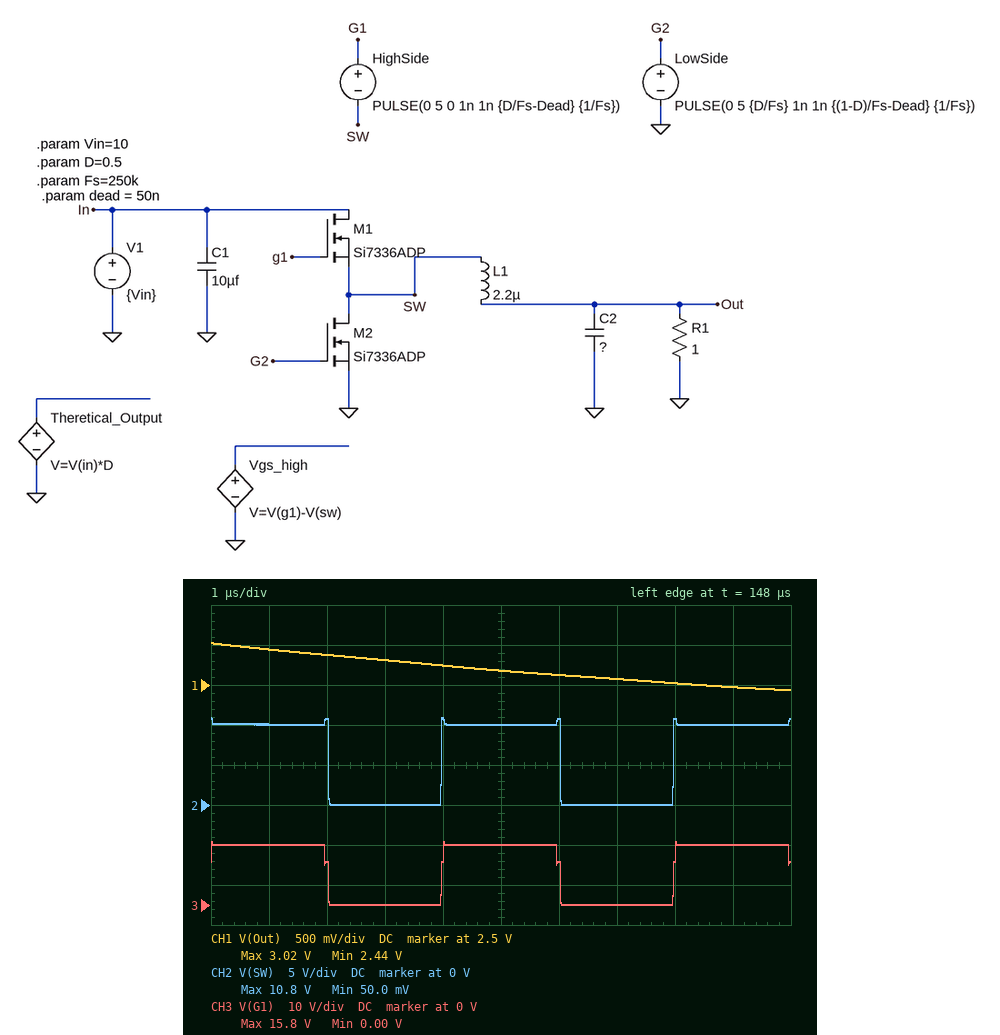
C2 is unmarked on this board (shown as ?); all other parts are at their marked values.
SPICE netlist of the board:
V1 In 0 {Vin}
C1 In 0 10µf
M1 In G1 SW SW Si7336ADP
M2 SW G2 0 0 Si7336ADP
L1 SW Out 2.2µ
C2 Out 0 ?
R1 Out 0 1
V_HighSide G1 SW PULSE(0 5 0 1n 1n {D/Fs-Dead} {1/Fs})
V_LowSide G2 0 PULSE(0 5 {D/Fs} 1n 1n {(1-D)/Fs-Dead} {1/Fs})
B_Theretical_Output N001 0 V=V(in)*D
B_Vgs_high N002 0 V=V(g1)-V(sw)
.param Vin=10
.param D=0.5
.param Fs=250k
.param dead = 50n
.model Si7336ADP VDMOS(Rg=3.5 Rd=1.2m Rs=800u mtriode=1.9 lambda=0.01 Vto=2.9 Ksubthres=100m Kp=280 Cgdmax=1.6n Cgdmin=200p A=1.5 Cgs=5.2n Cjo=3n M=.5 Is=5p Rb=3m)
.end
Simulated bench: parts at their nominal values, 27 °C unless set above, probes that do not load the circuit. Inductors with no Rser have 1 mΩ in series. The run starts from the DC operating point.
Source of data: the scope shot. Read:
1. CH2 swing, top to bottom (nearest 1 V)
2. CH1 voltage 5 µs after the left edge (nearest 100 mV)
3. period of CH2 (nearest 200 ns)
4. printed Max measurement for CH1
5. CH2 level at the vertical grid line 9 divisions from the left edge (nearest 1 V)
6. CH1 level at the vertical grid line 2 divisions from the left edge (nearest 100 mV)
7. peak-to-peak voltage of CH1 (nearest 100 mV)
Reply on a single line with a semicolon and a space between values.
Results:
11 V; 2.7 V; 4.0 µs; 3.02 V; 10 V; 2.9 V; 600 mV
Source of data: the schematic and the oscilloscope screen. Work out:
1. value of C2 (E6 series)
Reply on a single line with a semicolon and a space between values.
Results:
330 µF
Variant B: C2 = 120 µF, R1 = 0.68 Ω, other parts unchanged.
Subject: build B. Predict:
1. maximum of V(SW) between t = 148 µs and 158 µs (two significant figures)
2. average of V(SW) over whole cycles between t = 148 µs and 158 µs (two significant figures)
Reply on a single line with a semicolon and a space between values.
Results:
10 V; 4.8 V
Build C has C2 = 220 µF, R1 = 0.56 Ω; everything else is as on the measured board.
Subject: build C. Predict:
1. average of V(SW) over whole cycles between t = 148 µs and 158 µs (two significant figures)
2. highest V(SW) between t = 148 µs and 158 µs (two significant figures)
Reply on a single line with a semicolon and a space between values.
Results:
4.8 V; 10 V
